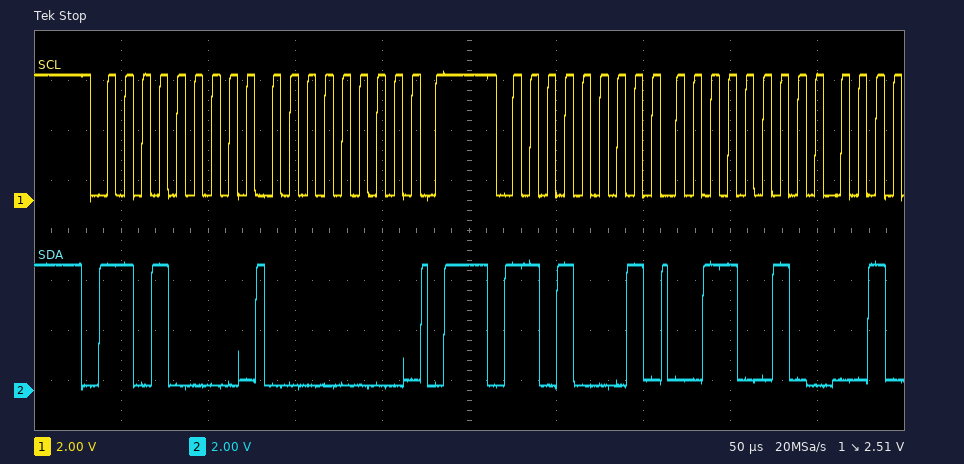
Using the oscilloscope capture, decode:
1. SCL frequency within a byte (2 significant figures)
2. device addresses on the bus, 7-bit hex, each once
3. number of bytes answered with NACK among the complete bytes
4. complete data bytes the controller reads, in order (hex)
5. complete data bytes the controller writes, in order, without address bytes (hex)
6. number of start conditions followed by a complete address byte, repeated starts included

100 kHz
0x68
0
32
00
2
